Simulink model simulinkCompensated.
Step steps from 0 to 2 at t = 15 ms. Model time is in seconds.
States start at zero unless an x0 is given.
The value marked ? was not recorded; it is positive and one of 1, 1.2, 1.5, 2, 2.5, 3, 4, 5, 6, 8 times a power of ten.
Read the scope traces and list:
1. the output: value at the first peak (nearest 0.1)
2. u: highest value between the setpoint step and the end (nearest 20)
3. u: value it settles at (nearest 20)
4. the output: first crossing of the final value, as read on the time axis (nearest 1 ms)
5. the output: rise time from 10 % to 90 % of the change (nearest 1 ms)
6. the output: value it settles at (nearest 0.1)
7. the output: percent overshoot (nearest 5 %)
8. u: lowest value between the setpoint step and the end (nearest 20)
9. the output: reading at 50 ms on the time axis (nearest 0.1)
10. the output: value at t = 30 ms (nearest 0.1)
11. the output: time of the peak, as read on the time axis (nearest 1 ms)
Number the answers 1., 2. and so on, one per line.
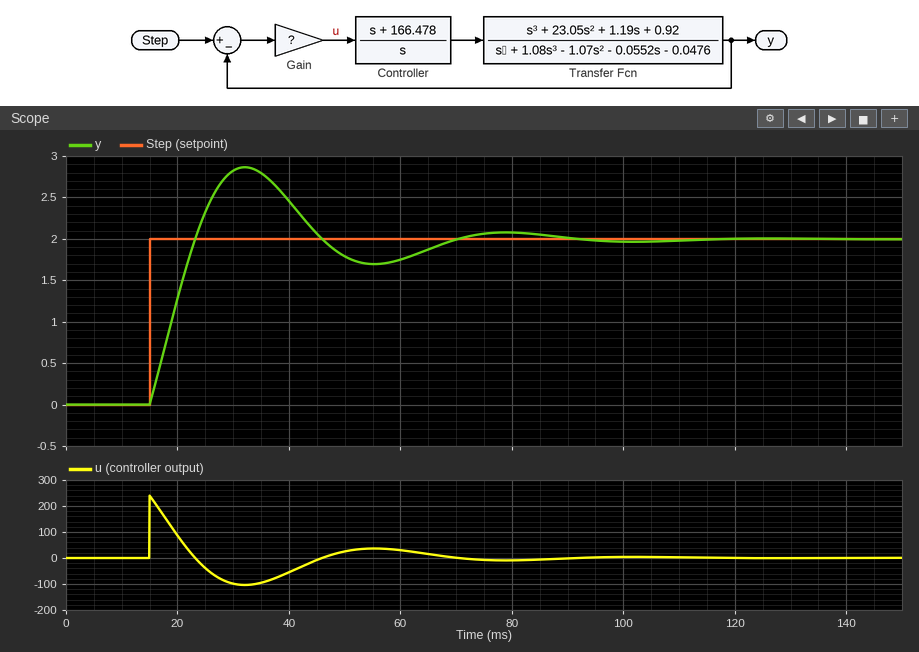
1. 2.9
2. 240
3. 0
4. 23 ms
5. 6 ms
6. 2.0
7. 45 %
8. -100
9. 1.8
10. 2.8
11. 32 ms
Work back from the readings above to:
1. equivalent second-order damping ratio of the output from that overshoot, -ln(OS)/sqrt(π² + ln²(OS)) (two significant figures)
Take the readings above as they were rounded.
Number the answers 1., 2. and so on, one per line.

1. 0.25
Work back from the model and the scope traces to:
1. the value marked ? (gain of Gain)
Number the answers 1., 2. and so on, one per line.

1. 120
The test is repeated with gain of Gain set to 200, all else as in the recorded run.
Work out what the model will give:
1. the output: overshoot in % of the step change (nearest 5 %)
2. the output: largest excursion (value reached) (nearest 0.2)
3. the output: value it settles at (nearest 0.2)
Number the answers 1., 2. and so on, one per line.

1. 35 %
2. 2.6
3. 2.0
